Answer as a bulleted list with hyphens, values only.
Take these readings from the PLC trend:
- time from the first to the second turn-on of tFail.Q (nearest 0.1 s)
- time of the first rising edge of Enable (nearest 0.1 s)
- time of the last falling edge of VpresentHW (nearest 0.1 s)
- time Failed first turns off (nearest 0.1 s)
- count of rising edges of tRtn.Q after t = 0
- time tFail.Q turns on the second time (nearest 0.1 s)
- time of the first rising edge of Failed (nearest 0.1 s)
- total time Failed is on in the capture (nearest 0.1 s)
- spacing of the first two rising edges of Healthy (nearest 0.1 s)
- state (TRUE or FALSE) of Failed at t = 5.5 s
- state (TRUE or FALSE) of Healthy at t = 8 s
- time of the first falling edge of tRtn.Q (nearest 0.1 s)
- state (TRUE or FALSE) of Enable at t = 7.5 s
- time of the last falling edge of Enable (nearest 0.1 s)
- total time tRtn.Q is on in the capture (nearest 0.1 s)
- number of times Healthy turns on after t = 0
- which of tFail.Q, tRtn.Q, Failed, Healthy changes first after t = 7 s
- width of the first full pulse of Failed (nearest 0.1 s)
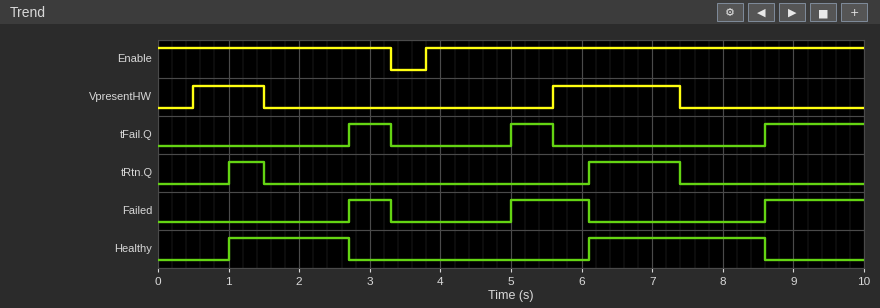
- 2.3 s
- 3.8 s
- 7.4 s
- 3.3 s
- 2
- 5.0 s
- 2.7 s
- 3.1 s
- 5.1 s
- TRUE
- TRUE
- 1.5 s
- TRUE
- 3.3 s
- 1.8 s
- 2
- tRtn.Q
- 0.6 s
